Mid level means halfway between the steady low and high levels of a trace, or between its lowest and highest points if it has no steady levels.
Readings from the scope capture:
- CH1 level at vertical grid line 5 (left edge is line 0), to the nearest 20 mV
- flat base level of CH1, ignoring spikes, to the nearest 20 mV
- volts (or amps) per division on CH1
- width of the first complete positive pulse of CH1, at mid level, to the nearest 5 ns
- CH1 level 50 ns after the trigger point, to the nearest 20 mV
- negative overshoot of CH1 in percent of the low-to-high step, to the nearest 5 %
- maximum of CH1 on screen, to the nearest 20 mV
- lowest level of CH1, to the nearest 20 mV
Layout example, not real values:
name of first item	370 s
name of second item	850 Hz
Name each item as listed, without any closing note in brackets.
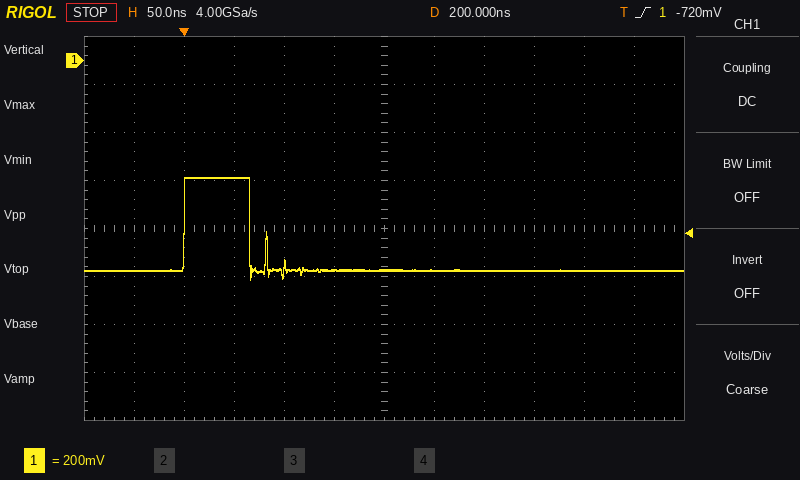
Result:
CH1 level at vertical grid line 5 (left edge is line 0), to the nearest 20 mV	-880 mV
flat base level of CH1, ignoring spikes, to the nearest 20 mV	-880 mV
volts (or amps) per division on CH1	200 mV
width of the first complete positive pulse of CH1, at mid level, to the nearest 5 ns	65 ns
CH1 level 50 ns after the trigger point, to the nearest 20 mV	-480 mV
negative overshoot of CH1 in percent of the low-to-high step, to the nearest 5 %	10 %
maximum of CH1 on screen, to the nearest 20 mV	-480 mV
lowest level of CH1, to the nearest 20 mV	-920 mV
